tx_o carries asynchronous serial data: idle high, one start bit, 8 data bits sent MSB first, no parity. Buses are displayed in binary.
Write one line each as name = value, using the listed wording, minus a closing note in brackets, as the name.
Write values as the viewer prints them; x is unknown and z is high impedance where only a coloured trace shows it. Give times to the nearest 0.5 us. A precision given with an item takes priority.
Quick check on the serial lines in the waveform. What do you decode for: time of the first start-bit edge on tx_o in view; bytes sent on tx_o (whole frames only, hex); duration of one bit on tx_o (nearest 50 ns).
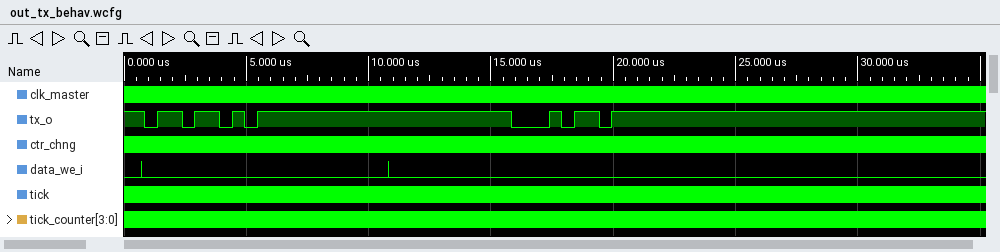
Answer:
time of the first start-bit edge on tx_o in view = 1 us
bytes sent on tx_o = DA, 2D
duration of one bit on tx_o = 500 ns
